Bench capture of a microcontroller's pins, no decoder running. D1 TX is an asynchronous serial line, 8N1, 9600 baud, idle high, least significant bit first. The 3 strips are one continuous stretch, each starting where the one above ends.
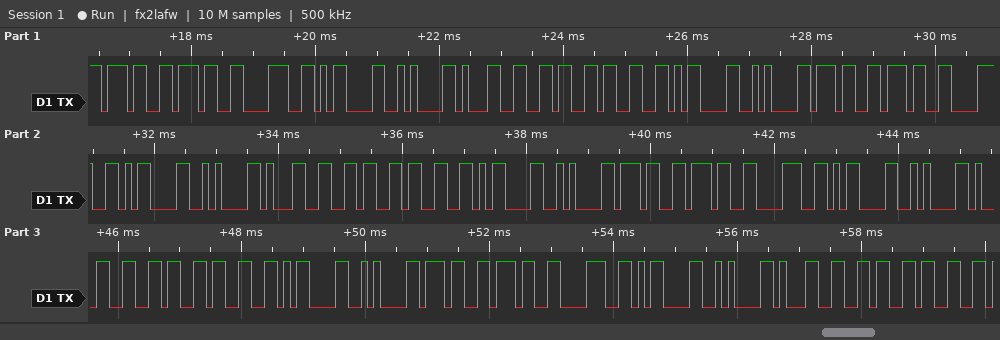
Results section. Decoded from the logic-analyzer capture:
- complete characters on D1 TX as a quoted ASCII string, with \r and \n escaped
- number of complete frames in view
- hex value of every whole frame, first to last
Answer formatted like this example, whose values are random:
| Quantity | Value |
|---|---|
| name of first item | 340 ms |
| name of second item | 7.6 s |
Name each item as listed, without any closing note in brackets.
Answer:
| Quantity | Value |
|---|---|
| complete characters on D1 TX as a quoted ASCII string, with \r and \n escaped | "778\r\n163\r\n778\r\n163\r\n778\r\n163\r\n778\r\n163" |
| number of complete frames in view | 38 |
| hex value of every whole frame, first to last | 37 37 38 0D 0A 31 36 33 0D 0A 37 37 38 0D 0A 31 36 33 0D 0A 37 37 38 0D 0A 31 36 33 0D 0A 37 37 38 0D 0A 31 36 33 |
